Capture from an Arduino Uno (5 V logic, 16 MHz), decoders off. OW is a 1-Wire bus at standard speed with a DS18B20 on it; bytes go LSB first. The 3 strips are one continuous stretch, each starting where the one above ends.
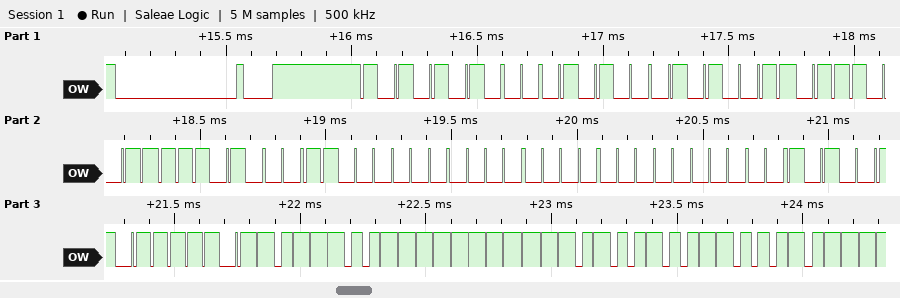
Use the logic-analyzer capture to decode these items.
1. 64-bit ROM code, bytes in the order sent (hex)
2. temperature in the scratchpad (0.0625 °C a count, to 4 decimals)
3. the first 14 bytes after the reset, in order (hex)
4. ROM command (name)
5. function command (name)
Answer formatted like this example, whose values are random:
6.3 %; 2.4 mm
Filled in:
28 CA CE 17 03 00 00 94; -6.1875 °C; 55 28 CA CE 17 03 00 00 94 BE 9D FF 4B 46; Match ROM; Read Scratchpad
